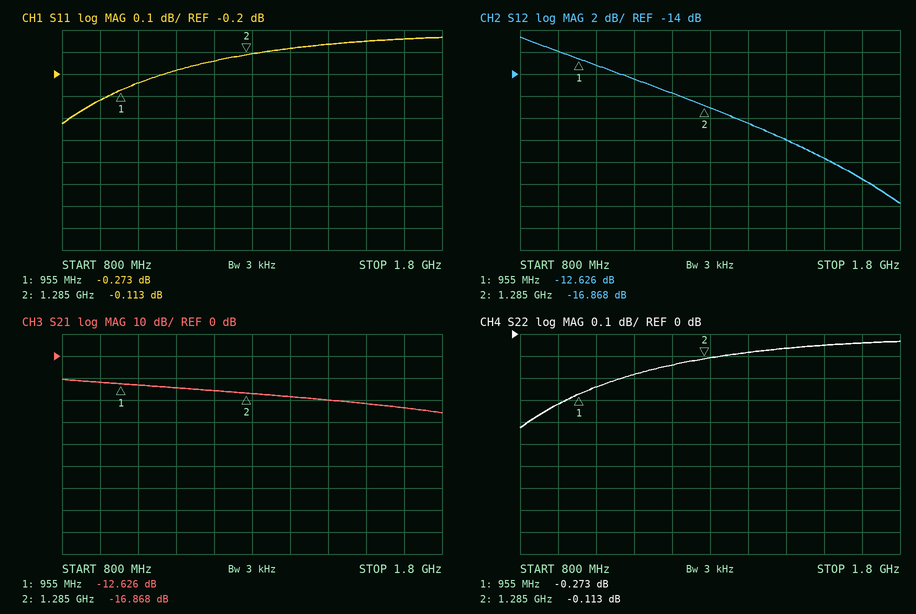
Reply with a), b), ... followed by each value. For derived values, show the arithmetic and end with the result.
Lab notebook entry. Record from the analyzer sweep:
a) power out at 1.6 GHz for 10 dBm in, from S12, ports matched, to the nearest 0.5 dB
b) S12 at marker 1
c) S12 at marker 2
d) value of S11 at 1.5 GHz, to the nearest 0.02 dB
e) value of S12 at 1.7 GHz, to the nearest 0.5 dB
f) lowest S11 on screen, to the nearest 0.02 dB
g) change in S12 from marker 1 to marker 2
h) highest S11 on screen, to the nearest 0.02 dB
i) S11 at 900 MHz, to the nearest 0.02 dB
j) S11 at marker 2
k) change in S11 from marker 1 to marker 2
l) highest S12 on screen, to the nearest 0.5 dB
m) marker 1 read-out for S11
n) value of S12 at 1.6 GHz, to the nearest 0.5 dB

a) 10 dBm + (-21.5 dB) = -11.5 dBm
b) -12.626 dB
c) -16.868 dB
d) -0.06 dB
e) -23.5 dB
f) -0.42 dB
g) -16.868 − (-12.626) = -4.242 dB
h) -0.04 dB
i) -0.32 dB
j) -0.113 dB
k) -0.113 − (-0.273) = 0.160 dB
l) -10.5 dB
m) -0.273 dB
n) -21.5 dB
